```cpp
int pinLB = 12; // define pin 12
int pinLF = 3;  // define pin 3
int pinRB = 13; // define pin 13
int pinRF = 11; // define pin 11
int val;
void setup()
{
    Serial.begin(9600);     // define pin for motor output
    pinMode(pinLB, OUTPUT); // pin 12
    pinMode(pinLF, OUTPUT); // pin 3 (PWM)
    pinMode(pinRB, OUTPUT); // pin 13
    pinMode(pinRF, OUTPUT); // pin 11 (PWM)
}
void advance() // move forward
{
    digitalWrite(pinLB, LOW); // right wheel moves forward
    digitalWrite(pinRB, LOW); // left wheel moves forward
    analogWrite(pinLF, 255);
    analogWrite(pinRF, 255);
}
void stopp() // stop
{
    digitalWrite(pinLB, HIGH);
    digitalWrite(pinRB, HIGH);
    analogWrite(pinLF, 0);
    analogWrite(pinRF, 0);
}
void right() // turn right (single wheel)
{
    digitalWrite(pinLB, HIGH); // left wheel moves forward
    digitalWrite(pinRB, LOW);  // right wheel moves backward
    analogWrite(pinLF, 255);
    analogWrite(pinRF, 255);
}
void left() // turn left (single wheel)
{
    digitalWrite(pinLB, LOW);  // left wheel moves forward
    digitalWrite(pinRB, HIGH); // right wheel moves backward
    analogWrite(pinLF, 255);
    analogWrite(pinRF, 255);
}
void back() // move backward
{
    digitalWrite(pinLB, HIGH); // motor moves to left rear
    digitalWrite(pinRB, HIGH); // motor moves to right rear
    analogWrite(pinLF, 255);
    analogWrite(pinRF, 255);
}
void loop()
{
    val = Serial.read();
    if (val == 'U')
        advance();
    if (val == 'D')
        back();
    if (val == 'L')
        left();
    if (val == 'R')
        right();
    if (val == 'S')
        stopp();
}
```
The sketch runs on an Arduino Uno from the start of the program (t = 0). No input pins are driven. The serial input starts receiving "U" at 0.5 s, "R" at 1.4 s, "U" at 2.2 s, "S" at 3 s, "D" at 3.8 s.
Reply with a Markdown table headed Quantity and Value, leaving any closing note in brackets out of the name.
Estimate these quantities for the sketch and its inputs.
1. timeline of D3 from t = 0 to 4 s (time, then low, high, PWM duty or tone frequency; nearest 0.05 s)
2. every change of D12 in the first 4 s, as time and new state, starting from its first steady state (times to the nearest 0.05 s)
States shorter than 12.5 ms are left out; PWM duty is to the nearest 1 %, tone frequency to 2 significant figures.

| Quantity | Value |
|---|---|
| timeline of D3 from t = 0 to 4 s | 0 s low; 0.5 s high; 3 s low; 3.8 s high |
| every change of D12 in the first 4 s, as time and new state, starting from its first steady state | 0 s low; 1.4 s high; 2.2 s low; 3 s high |
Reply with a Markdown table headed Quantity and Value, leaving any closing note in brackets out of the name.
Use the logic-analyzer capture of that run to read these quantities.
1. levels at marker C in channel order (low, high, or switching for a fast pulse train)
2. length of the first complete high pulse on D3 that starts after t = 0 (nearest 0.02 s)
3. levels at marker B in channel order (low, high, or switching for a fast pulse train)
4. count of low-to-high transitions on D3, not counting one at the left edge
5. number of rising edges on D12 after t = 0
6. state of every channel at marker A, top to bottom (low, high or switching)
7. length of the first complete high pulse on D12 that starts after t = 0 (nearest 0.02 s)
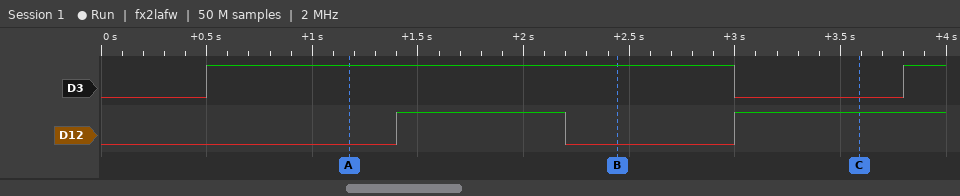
| Quantity | Value |
|---|---|
| levels at marker C in channel order | D3 low, D12 high |
| length of the first complete high pulse on D3 that starts after t = 0 | 2.50 s |
| levels at marker B in channel order | D3 high, D12 low |
| count of low-to-high transitions on D3, not counting one at the left edge | 2 |
| number of rising edges on D12 after t = 0 | 2 |
| state of every channel at marker A, top to bottom | D3 high, D12 low |
| length of the first complete high pulse on D12 that starts after t = 0 | 0.80 s |
